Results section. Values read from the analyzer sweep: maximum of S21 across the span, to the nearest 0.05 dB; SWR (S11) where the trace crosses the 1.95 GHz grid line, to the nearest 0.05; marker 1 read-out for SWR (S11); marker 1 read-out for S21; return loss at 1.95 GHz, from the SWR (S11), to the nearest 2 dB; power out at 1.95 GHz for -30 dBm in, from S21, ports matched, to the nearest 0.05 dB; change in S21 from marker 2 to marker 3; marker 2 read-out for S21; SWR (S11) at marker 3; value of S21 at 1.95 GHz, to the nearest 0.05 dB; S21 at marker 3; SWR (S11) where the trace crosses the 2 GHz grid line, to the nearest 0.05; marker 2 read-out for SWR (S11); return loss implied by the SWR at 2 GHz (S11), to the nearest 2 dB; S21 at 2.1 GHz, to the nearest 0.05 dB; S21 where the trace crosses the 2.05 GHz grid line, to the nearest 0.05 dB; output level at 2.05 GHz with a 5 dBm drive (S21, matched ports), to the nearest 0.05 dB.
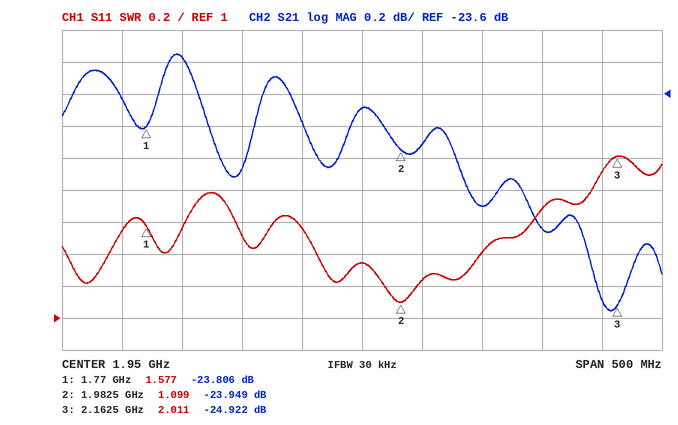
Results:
-23.35 dB
1.35
1.577
-23.806 dB
16 dB
-53.70 dBm
-0.973 dB
-23.949 dB
2.011
-23.70 dB
-24.922 dB
1.25
1.099
20 dB
-24.45 dB
-24.30 dB
-19.30 dBm
